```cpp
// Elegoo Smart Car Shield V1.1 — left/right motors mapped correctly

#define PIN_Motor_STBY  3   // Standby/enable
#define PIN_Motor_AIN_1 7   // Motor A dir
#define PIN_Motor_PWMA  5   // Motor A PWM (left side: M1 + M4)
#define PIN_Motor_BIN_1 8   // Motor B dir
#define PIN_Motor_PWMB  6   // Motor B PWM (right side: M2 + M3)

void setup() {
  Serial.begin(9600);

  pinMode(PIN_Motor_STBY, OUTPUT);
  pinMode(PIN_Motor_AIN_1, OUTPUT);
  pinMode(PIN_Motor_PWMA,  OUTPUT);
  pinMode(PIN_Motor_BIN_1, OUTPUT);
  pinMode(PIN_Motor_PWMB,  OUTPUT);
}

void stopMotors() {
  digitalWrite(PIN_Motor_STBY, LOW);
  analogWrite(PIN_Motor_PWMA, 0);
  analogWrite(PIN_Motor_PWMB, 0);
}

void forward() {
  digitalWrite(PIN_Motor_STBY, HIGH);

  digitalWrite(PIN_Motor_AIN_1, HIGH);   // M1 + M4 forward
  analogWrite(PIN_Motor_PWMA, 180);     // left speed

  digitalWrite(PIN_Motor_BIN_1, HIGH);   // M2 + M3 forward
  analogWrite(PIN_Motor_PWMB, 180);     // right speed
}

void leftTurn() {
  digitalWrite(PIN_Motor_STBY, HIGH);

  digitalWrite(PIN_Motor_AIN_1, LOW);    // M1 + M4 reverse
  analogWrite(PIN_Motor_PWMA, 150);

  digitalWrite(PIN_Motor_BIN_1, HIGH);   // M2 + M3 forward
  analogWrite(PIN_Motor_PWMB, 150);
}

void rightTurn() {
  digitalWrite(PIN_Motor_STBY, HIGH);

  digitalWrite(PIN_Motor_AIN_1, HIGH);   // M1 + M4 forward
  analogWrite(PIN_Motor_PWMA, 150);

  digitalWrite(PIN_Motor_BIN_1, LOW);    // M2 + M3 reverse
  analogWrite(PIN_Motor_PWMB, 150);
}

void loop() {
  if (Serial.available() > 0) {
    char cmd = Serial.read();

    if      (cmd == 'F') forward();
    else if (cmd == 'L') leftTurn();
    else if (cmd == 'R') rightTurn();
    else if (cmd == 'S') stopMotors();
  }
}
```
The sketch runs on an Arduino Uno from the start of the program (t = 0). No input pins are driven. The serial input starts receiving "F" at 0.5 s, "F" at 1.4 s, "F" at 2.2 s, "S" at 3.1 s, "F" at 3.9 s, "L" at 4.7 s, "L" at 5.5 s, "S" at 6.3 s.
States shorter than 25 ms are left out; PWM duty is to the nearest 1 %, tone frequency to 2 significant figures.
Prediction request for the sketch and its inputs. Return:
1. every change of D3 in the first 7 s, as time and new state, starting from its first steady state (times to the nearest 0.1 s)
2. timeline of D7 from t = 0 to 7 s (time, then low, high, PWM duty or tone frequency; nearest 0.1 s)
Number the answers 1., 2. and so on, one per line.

1. 0 s low; 0.5 s high; 3.1 s low; 3.9 s high; 6.3 s low
2. 0 s low; 0.5 s high; 4.7 s low
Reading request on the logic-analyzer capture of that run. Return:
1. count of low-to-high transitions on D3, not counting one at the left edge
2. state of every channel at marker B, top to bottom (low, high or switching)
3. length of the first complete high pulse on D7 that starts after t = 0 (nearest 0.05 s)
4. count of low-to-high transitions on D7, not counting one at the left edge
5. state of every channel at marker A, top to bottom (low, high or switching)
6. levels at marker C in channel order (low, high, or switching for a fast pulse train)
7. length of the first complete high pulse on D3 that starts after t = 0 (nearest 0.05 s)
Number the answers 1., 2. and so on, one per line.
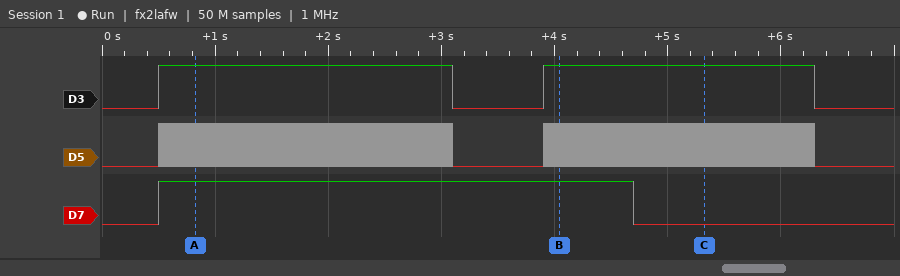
1. 2
2. D3 high, D5 switching, D7 high
3. 4.20 s
4. 1
5. D3 high, D5 switching, D7 high
6. D3 high, D5 switching, D7 low
7. 2.60 s
